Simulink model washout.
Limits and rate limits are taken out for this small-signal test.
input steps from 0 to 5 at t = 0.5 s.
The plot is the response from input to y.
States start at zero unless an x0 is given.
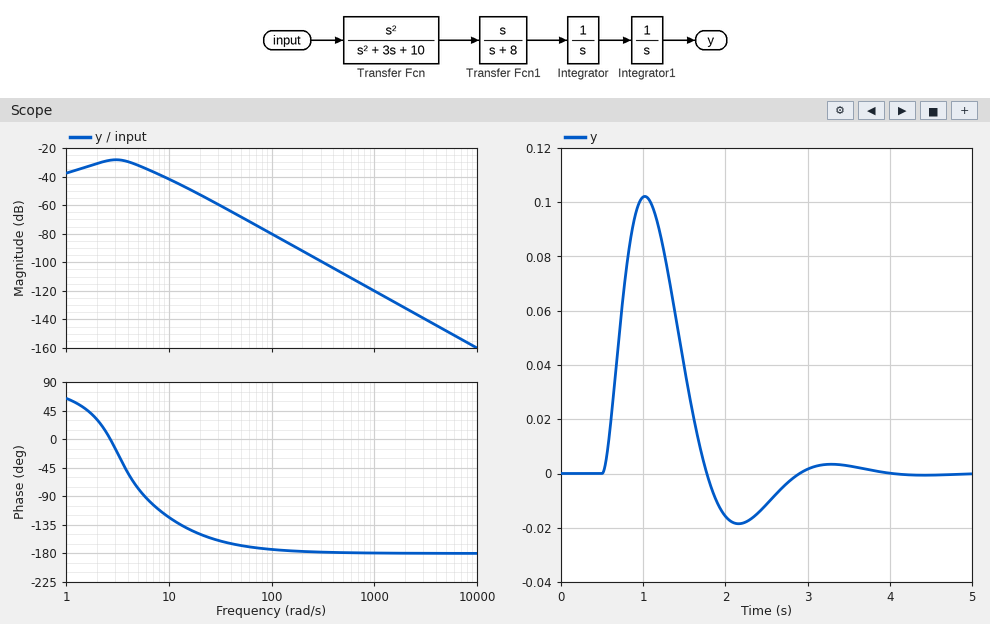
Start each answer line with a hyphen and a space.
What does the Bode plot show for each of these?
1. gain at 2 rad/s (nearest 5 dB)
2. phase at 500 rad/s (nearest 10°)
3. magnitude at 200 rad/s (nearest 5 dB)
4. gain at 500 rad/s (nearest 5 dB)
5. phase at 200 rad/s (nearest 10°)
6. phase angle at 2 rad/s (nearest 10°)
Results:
- -30 dB
- -180°
- -90 dB
- -110 dB
- -180°
- 30°
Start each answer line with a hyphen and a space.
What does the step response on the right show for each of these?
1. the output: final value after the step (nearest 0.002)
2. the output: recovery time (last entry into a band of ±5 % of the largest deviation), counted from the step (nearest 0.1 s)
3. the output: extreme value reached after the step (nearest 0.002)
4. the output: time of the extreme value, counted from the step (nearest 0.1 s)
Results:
- 0.000
- 2.2 s
- 0.102
- 0.5 s
